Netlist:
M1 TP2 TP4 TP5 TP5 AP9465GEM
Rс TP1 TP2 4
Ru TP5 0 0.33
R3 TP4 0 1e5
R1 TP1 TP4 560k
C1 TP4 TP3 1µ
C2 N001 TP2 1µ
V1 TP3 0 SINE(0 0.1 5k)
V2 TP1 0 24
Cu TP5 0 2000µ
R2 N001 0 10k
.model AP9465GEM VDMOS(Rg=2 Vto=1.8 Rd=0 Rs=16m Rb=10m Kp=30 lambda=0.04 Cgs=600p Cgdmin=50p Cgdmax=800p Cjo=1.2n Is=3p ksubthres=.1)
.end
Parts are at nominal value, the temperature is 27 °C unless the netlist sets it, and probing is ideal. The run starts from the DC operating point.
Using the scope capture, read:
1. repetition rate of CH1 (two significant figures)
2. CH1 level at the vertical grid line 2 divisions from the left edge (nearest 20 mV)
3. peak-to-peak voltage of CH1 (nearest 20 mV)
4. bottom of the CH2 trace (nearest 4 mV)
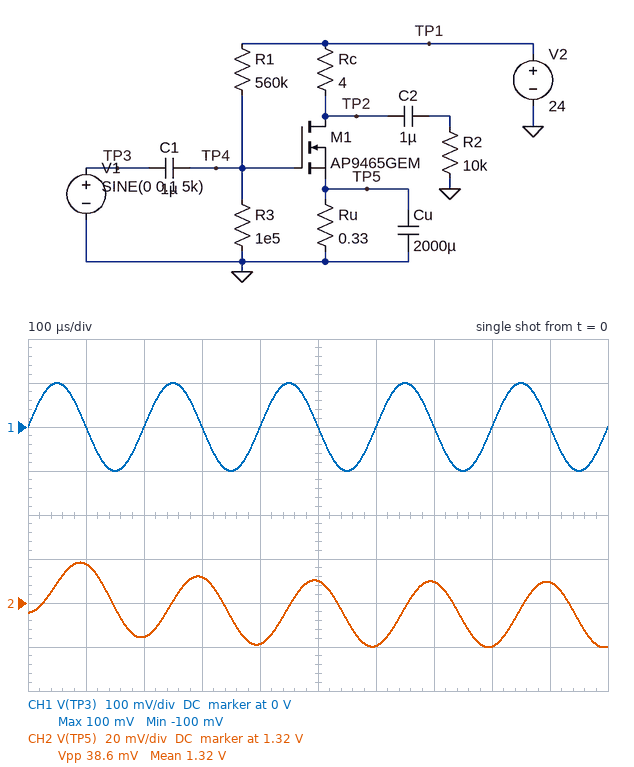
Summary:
5.0 kHz
0 V
200 mV
1.300 V
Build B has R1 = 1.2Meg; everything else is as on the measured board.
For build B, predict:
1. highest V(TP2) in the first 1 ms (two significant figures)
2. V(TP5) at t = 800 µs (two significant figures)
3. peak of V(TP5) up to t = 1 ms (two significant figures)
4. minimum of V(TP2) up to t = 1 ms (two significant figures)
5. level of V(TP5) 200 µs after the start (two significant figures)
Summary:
24 V
51 mV
58 mV
22 V
48 mV
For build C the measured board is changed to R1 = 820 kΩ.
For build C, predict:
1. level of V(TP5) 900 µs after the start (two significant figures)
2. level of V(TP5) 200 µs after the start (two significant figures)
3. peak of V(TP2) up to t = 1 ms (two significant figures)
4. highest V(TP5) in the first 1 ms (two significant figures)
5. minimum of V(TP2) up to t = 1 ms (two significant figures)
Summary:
550 mV
530 mV
21 V
560 mV
14 V
